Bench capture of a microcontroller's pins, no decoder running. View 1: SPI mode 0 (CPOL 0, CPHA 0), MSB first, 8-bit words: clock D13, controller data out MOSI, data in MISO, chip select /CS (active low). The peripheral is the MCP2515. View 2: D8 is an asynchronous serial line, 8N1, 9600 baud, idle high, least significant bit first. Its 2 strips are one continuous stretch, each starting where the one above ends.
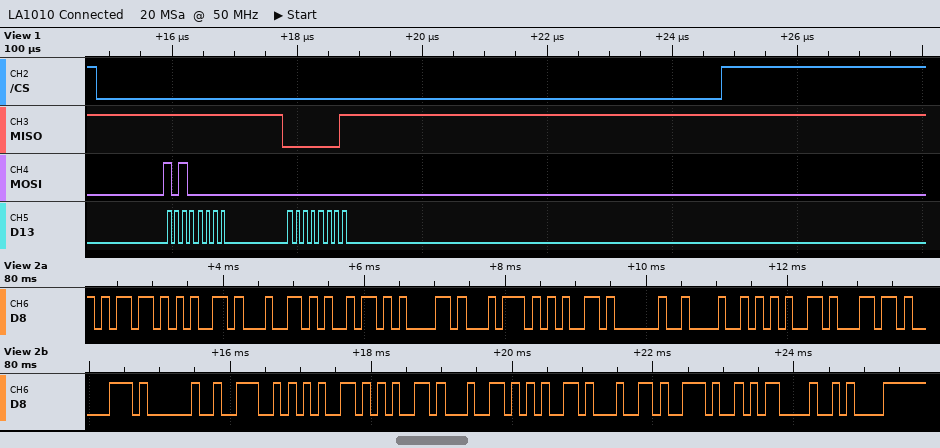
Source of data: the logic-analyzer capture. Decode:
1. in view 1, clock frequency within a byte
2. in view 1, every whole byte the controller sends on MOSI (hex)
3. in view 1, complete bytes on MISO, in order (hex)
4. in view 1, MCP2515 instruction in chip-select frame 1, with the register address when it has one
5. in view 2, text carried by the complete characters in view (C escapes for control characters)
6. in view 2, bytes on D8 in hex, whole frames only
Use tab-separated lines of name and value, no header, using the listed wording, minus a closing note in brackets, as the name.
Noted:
in view 1, clock frequency within a byte	8 MHz
in view 1, every whole byte the controller sends on MOSI	0xA0 0x00
in view 1, complete bytes on MISO, in order	0xFF 0x01
in view 1, MCP2515 instruction in chip-select frame 1, with the register address when it has one	READ STATUS
in view 2, text carried by the complete characters in view	"mediate Help Needed.\r\n"
in view 2, bytes on D8 in hex, whole frames only	0x6D 0x65 0x64 0x69 0x61 0x74 0x65 0x20 0x48 0x65 0x6C 0x70 0x20 0x4E 0x65 0x65 0x64 0x65 0x64 0x2E 0x0D 0x0A
